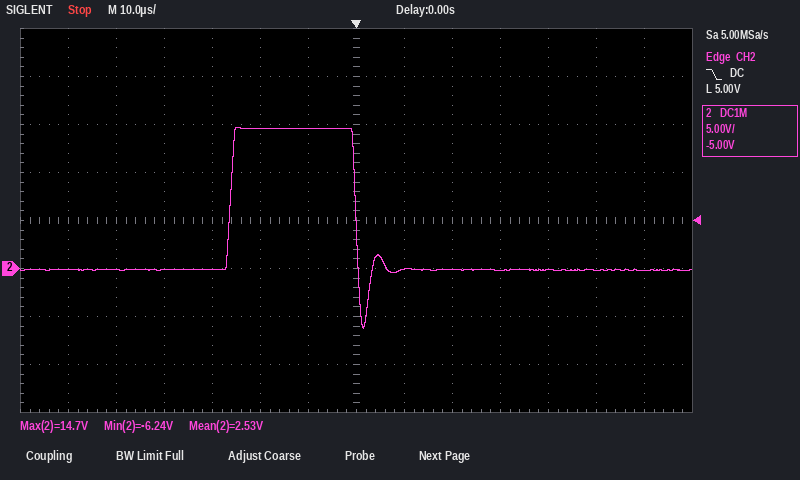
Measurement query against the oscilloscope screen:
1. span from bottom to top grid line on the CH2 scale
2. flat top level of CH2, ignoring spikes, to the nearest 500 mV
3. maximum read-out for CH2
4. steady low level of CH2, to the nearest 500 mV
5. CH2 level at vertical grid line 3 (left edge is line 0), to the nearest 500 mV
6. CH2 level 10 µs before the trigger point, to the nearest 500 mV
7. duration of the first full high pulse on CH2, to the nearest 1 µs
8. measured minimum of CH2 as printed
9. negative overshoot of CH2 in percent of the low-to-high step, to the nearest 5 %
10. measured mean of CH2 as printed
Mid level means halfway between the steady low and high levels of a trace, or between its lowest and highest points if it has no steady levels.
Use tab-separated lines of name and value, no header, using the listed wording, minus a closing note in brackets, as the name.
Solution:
span from bottom to top grid line on the CH2 scale	40 V
flat top level of CH2, ignoring spikes, to the nearest 500 mV	14.5 V
maximum read-out for CH2	14.7 V
steady low level of CH2, to the nearest 500 mV	0.0 V
CH2 level at vertical grid line 3 (left edge is line 0), to the nearest 500 mV	0.0 V
CH2 level 10 µs before the trigger point, to the nearest 500 mV	14.5 V
duration of the first full high pulse on CH2, to the nearest 1 µs	26 µs
measured minimum of CH2 as printed	-6.24 V
negative overshoot of CH2 in percent of the low-to-high step, to the nearest 5 %	40 %
measured mean of CH2 as printed	2.53 V
